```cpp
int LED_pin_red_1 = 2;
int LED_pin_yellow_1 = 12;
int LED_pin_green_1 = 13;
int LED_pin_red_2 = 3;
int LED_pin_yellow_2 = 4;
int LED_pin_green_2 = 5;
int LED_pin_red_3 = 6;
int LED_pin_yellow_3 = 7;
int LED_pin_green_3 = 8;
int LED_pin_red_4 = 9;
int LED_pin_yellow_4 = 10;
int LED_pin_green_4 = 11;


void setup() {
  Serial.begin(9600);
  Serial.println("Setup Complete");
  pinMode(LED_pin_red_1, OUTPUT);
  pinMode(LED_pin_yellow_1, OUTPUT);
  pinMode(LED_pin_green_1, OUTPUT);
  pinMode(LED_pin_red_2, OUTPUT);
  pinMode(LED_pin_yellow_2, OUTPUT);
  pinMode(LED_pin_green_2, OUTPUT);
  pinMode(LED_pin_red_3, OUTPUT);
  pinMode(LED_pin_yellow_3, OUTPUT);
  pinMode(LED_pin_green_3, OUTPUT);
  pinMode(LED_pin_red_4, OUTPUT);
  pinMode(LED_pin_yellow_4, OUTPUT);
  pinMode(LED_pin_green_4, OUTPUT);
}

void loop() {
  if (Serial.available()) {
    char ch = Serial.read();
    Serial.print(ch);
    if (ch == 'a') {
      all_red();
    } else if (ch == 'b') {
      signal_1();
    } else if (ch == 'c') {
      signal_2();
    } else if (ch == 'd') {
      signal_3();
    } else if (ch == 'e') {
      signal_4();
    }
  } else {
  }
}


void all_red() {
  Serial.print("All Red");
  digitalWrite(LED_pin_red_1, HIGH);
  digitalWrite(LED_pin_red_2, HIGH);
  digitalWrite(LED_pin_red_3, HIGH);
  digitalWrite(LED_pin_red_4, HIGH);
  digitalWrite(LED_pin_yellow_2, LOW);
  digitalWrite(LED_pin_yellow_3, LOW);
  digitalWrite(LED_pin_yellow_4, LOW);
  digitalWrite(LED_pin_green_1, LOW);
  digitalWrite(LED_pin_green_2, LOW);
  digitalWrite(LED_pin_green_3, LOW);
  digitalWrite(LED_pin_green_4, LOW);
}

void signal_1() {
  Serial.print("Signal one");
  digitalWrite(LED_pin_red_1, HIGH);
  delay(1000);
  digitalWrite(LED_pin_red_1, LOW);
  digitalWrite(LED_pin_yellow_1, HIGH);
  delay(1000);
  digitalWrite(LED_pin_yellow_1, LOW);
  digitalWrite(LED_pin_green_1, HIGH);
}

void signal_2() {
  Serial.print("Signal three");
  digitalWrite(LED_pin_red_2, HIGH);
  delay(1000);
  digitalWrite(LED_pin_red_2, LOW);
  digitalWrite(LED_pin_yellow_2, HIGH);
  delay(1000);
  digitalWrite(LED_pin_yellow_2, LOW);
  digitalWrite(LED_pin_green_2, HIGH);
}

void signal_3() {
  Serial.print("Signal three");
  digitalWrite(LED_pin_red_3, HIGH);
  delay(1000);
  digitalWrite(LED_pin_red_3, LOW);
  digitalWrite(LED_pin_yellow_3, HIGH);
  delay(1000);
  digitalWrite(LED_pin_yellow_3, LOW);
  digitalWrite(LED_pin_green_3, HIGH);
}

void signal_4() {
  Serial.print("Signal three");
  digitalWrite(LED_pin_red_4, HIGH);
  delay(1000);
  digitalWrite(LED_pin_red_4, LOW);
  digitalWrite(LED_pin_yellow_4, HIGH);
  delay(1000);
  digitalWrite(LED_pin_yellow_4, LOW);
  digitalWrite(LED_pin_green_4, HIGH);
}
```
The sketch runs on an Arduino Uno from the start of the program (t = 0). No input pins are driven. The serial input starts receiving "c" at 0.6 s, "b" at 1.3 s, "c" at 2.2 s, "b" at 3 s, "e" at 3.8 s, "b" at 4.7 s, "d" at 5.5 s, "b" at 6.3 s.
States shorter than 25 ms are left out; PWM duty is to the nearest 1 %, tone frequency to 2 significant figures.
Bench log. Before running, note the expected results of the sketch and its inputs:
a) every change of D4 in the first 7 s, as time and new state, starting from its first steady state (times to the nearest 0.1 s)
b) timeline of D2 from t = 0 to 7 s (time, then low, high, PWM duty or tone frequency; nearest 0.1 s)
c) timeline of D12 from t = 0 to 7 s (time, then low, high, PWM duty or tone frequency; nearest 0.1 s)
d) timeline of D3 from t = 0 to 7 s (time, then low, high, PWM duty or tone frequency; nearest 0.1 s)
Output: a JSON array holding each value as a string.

["0 s low; 1.6 s high; 2.6 s low; 5.6 s high; 6.6 s low", "0 s low; 2.6 s high; 3.6 s low; 6.6 s high", "0 s low; 3.6 s high; 4.6 s low", "0 s low; 0.6 s high; 1.6 s low; 4.6 s high; 5.6 s low"]
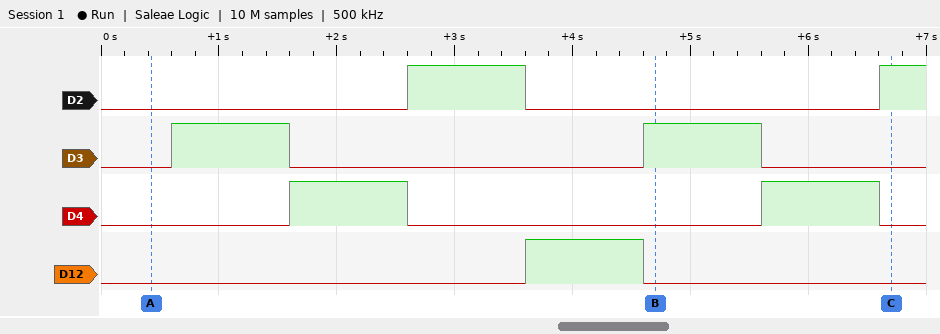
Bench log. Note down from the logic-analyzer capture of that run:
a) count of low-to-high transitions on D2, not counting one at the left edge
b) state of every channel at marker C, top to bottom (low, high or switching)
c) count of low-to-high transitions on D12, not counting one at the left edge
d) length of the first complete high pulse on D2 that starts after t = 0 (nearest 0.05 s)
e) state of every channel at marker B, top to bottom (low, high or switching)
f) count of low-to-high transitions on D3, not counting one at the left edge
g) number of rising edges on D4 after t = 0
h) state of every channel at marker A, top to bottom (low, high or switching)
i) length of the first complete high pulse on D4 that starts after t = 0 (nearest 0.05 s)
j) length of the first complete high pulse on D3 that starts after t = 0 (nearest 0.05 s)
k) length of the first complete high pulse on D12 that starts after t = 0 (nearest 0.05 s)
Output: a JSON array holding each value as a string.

["2", "D2 high, D3 low, D4 low, D12 low", "1", "1.00 s", "D2 low, D3 high, D4 low, D12 low", "2", "2", "D2 low, D3 low, D4 low, D12 low", "1.00 s", "1.00 s", "1.00 s"]
